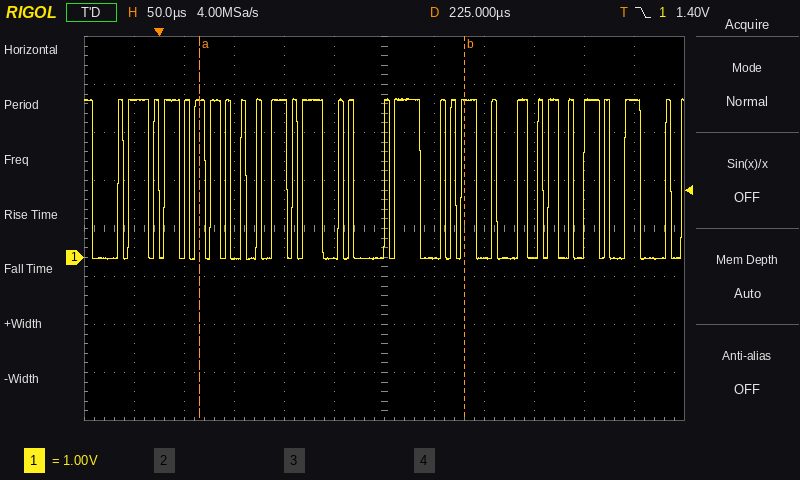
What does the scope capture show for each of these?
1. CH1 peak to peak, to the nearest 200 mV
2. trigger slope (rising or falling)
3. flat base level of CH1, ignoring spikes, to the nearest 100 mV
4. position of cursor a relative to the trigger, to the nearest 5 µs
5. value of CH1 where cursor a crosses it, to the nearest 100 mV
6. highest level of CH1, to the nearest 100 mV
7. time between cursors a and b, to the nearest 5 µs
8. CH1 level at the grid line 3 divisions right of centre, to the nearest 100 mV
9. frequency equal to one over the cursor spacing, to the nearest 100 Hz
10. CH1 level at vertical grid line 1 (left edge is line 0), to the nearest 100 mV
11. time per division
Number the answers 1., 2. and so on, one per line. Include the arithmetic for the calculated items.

1. 3.4 V
2. falling
3. 0.0 V
4. +40 µs
5. 3.3 V
6. 3.3 V
7. 265 µs
8. 0.0 V
9. 1 / 265 µs ≈ 3.8 kHz
10. 3.3 V
11. 50 µs
